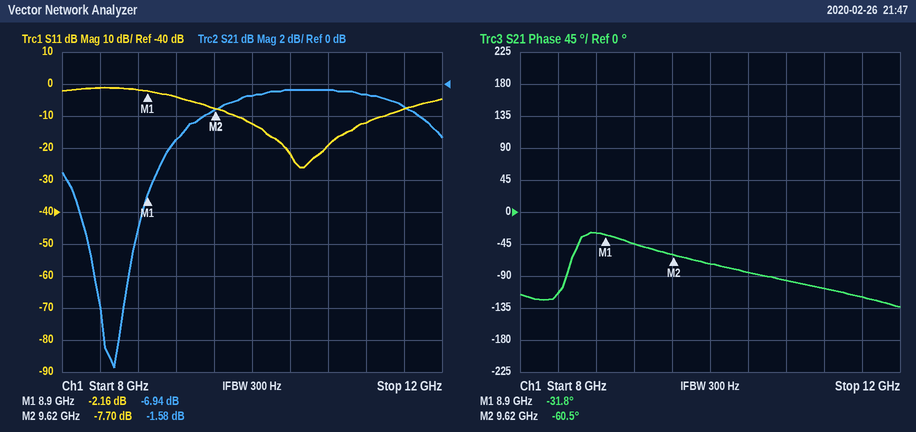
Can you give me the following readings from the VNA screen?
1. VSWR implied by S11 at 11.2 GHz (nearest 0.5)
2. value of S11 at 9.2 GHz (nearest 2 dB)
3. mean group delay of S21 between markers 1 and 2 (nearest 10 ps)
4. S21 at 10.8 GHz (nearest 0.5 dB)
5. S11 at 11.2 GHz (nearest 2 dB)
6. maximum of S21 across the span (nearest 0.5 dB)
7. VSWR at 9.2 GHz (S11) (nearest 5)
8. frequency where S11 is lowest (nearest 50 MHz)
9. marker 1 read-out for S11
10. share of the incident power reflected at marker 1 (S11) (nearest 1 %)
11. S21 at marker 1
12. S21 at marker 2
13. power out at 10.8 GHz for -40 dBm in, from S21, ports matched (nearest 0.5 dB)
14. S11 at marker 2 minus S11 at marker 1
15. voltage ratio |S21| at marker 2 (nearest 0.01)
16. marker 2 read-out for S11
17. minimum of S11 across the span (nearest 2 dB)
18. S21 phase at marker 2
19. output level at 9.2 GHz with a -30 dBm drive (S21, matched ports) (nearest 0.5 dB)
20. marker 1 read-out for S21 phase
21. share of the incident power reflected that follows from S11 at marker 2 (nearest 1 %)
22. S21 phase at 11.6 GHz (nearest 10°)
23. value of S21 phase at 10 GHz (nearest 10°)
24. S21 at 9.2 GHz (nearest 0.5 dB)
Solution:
1.5
-4 dB
110 ps
-0.5 dB
-12 dB
-0.5 dB
5
10.50 GHz
-2.16 dB
61 %
-6.94 dB
-1.58 dB
-40.5 dBm
-5.54 dB
0.83
-7.70 dB
-26 dB
-60.5°
-33.5 dBm
-31.8°
17 %
-120°
-70°
-3.5 dB
